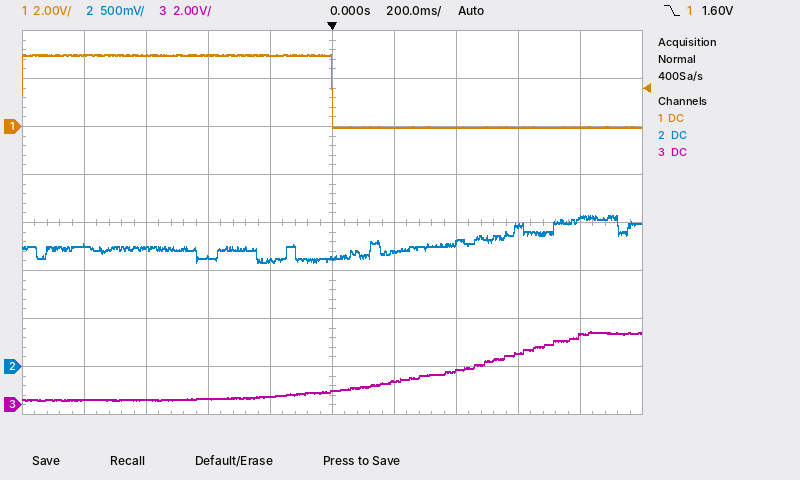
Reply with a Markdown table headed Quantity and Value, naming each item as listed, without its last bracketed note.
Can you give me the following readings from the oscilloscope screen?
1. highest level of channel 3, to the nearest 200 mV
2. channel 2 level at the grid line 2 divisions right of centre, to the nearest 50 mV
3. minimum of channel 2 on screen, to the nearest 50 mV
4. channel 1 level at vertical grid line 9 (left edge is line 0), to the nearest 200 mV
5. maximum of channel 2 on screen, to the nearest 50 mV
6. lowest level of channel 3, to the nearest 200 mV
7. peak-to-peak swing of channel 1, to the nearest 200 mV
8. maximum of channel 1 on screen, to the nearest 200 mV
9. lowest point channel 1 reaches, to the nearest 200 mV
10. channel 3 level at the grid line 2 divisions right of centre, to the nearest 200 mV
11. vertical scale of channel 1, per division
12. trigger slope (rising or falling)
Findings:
| Quantity | Value |
|---|---|
| highest level of channel 3, to the nearest 200 mV | 3.0 V |
| channel 2 level at the grid line 2 divisions right of centre, to the nearest 50 mV | 1.30 V |
| minimum of channel 2 on screen, to the nearest 50 mV | 1.10 V |
| channel 1 level at vertical grid line 9 (left edge is line 0), to the nearest 200 mV | 0.0 V |
| maximum of channel 2 on screen, to the nearest 50 mV | 1.55 V |
| lowest level of channel 3, to the nearest 200 mV | 200 mV |
| peak-to-peak swing of channel 1, to the nearest 200 mV | 3.0 V |
| maximum of channel 1 on screen, to the nearest 200 mV | 3.0 V |
| lowest point channel 1 reaches, to the nearest 200 mV | 0.0 V |
| channel 3 level at the grid line 2 divisions right of centre, to the nearest 200 mV | 1.4 V |
| vertical scale of channel 1, per division | 2 V |
| trigger slope | falling |
